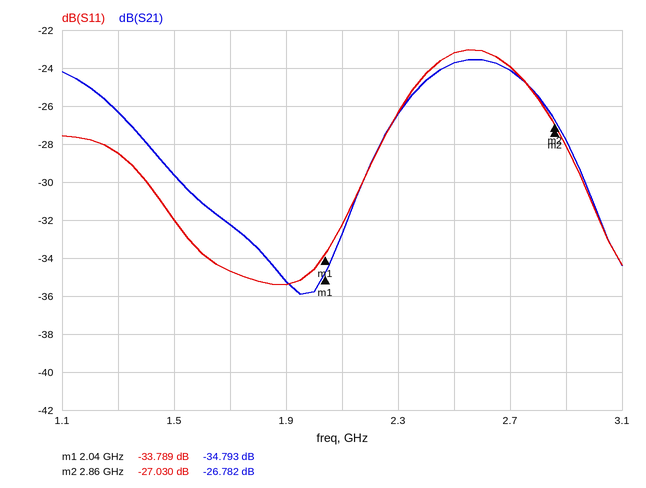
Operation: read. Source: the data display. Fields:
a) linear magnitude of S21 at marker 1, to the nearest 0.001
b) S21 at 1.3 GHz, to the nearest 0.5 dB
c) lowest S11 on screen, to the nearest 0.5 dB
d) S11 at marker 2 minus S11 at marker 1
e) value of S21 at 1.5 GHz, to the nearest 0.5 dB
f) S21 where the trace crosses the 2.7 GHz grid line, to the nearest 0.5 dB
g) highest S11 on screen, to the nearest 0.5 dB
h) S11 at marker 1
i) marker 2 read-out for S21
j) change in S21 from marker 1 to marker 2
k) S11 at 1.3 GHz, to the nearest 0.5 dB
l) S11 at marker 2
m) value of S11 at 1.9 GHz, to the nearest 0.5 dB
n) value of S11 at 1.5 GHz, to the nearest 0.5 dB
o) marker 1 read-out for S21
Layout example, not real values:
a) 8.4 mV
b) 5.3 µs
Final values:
a) 0.018
b) -26.5 dB
c) -35.5 dB
d) 6.759 dB
e) -29.5 dB
f) -24.0 dB
g) -23.0 dB
h) -33.789 dB
i) -26.782 dB
j) 8.011 dB
k) -28.5 dB
l) -27.030 dB
m) -35.5 dB
n) -32.0 dB
o) -34.793 dB
